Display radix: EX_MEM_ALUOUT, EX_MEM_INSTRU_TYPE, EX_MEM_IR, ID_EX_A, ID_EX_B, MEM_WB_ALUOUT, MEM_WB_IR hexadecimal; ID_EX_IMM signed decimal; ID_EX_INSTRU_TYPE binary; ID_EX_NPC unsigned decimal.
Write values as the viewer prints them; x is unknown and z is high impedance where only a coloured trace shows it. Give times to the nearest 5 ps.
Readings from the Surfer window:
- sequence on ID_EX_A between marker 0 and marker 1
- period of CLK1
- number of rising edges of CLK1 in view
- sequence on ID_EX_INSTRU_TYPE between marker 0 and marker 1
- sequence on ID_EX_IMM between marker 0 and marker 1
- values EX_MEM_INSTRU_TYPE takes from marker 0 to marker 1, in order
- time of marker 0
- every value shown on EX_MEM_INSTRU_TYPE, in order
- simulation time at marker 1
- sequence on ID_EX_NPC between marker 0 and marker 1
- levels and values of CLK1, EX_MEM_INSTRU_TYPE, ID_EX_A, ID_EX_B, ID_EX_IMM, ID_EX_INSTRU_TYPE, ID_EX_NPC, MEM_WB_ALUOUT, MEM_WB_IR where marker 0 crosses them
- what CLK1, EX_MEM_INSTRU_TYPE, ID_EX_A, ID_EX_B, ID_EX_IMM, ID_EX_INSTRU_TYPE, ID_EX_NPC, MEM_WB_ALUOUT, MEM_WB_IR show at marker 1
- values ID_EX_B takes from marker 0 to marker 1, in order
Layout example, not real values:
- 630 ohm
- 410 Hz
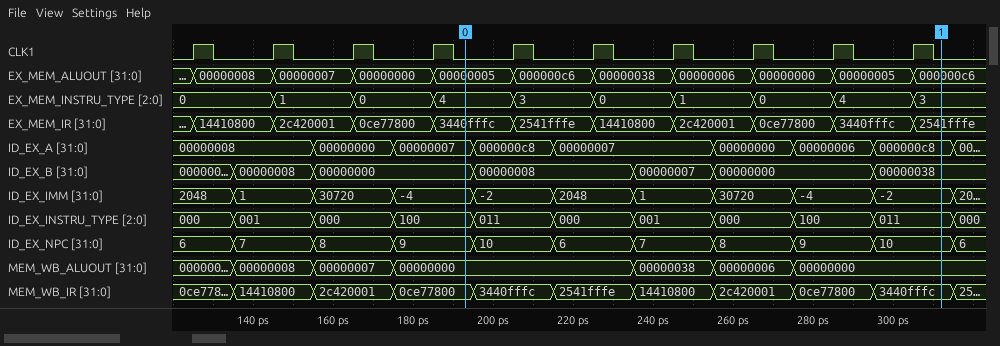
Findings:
- 00000007, 000000c8, 00000007, 00000000, 00000006, 000000c8
- 20 ps
- 10
- 100, 011, 000, 001, 000, 100, 011
- -4, -2, 2048, 1, 30720, -4, -2
- 4, 3, 0, 1, 0, 4, 3
- 195 ps
- 0, 1, 0, 4, 3, 0, 1, 0, 4, 3
- 310 ps
- 9, 10, 6, 7, 8, 9, 10
- CLK1=0, EX_MEM_INSTRU_TYPE=4, ID_EX_A=00000007, ID_EX_B=00000000, ID_EX_IMM=-4, ID_EX_INSTRU_TYPE=100, ID_EX_NPC=9, MEM_WB_ALUOUT=00000000, MEM_WB_IR=0ce77800
- CLK1=0, EX_MEM_INSTRU_TYPE=3, ID_EX_A=000000c8, ID_EX_B=00000038, ID_EX_IMM=-2, ID_EX_INSTRU_TYPE=011, ID_EX_NPC=10, MEM_WB_ALUOUT=00000000, MEM_WB_IR=3440fffc
- 00000000, 00000008, 00000007, 00000000, 00000038
